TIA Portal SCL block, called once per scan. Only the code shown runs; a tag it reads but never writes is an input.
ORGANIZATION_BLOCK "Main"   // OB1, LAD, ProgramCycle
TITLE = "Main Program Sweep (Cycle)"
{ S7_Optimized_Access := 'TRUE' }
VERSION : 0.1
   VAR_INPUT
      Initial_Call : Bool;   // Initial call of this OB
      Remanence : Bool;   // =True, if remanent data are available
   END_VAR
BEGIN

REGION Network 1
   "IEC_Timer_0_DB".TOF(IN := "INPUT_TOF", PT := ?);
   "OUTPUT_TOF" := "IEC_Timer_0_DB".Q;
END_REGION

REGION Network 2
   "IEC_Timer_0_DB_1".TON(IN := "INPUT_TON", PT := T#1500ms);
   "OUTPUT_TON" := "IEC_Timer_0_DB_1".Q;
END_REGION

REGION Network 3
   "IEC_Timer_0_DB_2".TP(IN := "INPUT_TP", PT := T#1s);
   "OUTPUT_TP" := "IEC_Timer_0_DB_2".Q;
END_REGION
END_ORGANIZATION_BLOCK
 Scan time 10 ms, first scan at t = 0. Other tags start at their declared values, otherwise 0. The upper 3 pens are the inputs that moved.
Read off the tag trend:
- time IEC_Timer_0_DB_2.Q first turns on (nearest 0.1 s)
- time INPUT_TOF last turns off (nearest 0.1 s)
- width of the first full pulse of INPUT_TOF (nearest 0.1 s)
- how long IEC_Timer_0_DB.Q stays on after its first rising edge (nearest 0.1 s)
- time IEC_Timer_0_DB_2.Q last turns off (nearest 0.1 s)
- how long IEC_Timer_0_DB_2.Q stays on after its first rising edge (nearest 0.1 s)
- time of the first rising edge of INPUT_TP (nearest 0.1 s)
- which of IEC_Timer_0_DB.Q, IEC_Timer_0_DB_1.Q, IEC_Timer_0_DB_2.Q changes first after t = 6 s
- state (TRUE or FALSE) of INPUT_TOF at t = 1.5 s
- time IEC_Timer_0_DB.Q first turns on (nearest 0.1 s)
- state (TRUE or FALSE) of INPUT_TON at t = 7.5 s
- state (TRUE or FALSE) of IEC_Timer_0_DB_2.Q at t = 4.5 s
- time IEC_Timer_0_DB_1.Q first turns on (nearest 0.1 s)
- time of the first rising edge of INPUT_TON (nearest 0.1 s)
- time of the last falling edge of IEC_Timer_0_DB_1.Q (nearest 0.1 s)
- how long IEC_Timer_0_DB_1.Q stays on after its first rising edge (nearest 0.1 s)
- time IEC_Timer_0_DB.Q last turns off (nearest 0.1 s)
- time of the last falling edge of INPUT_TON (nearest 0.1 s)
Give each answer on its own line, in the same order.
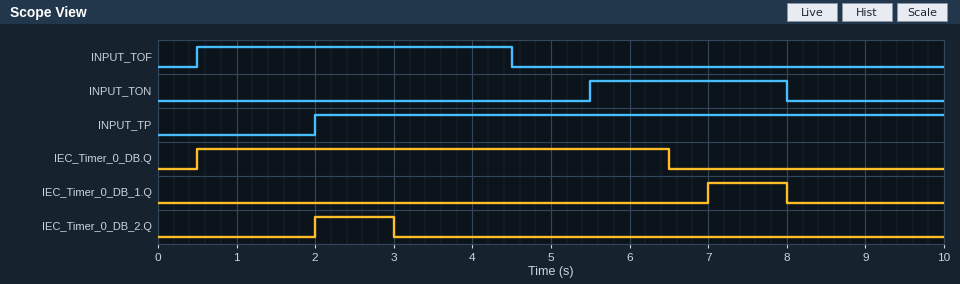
2.0 s
4.5 s
4.0 s
6.0 s
3.0 s
1.0 s
2.0 s
IEC_Timer_0_DB.Q
TRUE
0.5 s
TRUE
FALSE
7.0 s
5.5 s
8.0 s
1.0 s
6.5 s
8.0 s
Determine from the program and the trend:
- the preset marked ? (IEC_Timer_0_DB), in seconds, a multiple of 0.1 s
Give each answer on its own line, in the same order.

2.0 s
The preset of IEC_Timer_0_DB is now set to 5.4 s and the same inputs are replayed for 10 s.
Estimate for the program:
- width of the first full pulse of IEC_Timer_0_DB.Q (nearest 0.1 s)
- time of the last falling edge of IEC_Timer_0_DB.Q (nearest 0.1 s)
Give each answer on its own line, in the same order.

9.4 s
9.9 s
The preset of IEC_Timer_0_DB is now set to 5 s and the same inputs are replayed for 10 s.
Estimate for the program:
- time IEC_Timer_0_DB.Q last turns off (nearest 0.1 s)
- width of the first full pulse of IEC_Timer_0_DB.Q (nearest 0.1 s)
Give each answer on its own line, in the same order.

9.5 s
9.0 s
